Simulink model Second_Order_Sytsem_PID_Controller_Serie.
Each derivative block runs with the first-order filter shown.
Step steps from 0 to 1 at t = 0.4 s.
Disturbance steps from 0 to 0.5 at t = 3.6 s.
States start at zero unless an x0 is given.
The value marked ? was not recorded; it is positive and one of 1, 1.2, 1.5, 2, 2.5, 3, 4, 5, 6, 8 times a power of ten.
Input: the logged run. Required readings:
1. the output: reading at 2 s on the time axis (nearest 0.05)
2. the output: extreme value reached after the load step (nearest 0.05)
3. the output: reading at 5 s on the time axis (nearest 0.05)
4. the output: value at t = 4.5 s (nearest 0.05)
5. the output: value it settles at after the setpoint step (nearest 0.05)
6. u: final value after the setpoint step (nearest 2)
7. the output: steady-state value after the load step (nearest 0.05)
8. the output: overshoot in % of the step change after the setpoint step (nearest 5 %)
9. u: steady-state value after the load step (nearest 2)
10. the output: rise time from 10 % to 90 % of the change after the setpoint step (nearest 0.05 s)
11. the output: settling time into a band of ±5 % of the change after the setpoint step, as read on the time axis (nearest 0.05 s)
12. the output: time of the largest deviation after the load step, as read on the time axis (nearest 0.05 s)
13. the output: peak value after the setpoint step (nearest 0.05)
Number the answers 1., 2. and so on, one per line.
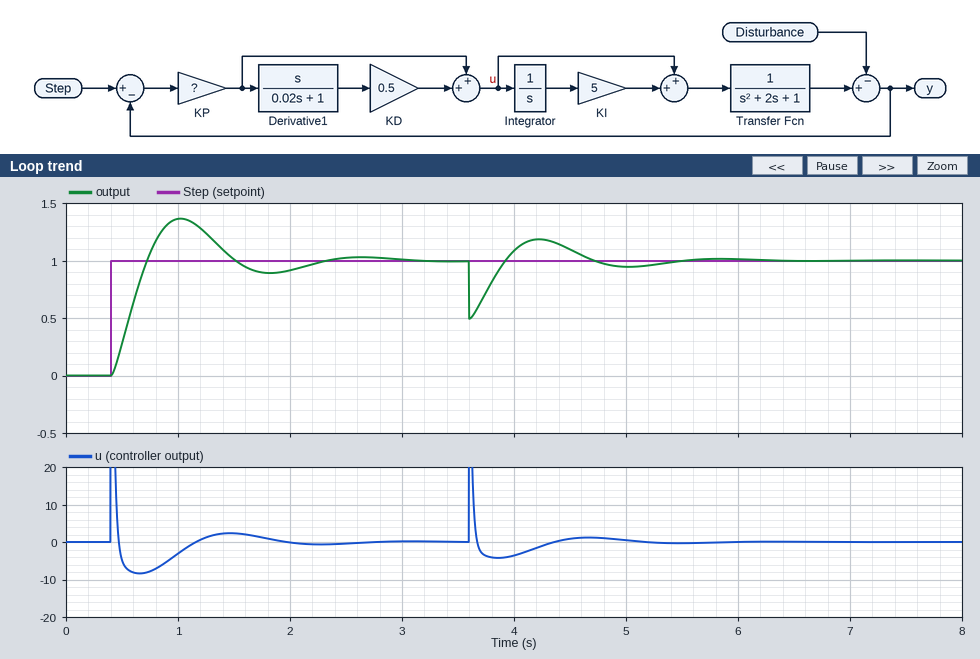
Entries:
1. 0.90
2. 0.50
3. 0.95
4. 1.10
5. 1.00
6. 0
7. 1.00
8. 35 %
9. 0
10. 0.25 s
11. 2.15 s
12. 3.60 s
13. 1.35
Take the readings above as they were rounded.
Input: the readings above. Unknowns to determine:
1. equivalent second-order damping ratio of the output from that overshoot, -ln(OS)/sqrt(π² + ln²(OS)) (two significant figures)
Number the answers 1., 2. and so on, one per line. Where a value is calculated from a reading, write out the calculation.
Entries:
1. ln(0.35) = -1.050; 1.050 / sqrt(9.870 + 1.102) = 0.32
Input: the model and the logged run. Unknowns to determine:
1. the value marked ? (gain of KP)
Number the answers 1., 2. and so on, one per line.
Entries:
1. 6
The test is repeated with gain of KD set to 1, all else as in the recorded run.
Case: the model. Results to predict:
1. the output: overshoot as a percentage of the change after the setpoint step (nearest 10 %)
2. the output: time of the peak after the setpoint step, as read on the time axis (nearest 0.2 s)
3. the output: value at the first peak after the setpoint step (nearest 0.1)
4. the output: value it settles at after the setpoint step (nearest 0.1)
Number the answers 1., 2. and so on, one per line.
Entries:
1. 20 %
2. 0.8 s
3. 1.2
4. 1.0
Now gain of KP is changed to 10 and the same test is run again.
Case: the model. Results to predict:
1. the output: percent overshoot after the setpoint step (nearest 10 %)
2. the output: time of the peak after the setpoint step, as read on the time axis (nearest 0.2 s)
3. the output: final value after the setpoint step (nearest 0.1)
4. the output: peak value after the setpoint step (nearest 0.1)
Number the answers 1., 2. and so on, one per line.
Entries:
1. 30 %
2. 0.8 s
3. 1.0
4. 1.3
